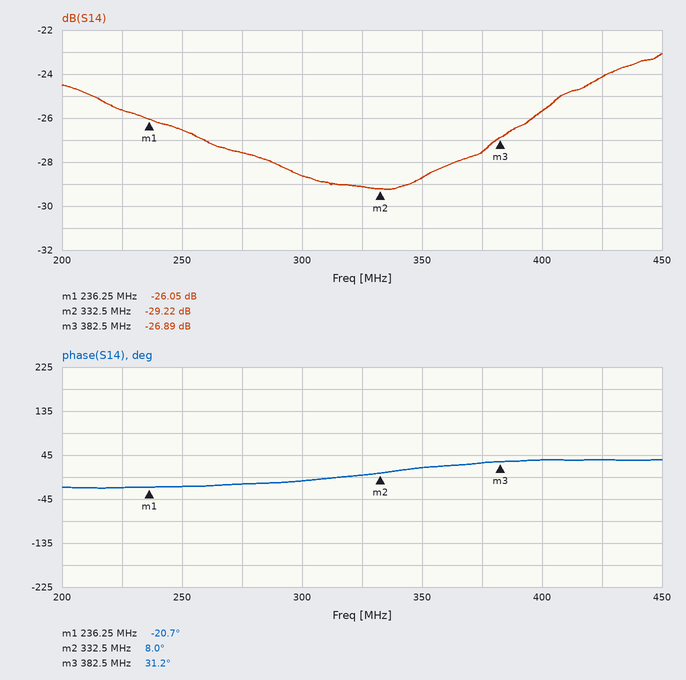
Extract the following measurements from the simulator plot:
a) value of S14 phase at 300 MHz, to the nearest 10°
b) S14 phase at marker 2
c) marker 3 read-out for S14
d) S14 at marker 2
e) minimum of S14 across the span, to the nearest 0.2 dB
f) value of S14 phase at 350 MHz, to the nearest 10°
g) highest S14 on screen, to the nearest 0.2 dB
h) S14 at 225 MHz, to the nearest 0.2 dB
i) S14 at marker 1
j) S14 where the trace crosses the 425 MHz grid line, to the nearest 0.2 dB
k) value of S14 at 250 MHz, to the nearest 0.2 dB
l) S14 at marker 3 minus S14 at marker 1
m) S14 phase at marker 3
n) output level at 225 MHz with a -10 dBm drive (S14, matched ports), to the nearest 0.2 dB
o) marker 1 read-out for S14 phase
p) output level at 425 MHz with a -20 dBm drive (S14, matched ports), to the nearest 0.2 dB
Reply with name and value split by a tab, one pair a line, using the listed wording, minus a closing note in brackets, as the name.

value of S14 phase at 300 MHz, to the nearest 10°	-10°
S14 phase at marker 2	8.0°
marker 3 read-out for S14	-26.89 dB
S14 at marker 2	-29.22 dB
minimum of S14 across the span, to the nearest 0.2 dB	-29.2 dB
value of S14 phase at 350 MHz, to the nearest 10°	20°
highest S14 on screen, to the nearest 0.2 dB	-23.0 dB
S14 at 225 MHz, to the nearest 0.2 dB	-25.6 dB
S14 at marker 1	-26.05 dB
S14 where the trace crosses the 425 MHz grid line, to the nearest 0.2 dB	-24.2 dB
value of S14 at 250 MHz, to the nearest 0.2 dB	-26.6 dB
S14 at marker 3 minus S14 at marker 1	-0.84 dB
S14 phase at marker 3	31.2°
output level at 225 MHz with a -10 dBm drive (S14, matched ports), to the nearest 0.2 dB	-35.6 dBm
marker 1 read-out for S14 phase	-20.7°
output level at 425 MHz with a -20 dBm drive (S14, matched ports), to the nearest 0.2 dB	-44.2 dBm
